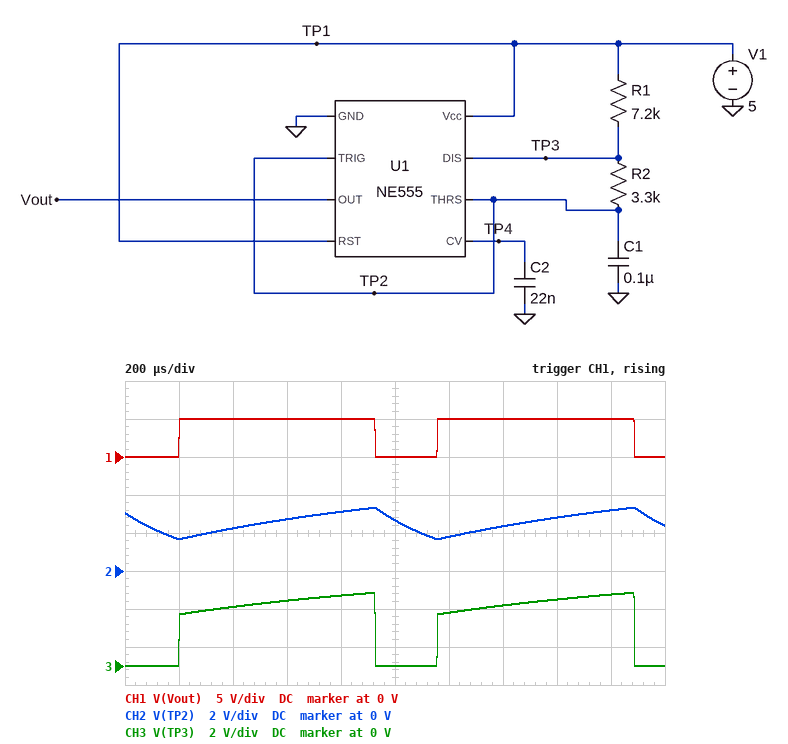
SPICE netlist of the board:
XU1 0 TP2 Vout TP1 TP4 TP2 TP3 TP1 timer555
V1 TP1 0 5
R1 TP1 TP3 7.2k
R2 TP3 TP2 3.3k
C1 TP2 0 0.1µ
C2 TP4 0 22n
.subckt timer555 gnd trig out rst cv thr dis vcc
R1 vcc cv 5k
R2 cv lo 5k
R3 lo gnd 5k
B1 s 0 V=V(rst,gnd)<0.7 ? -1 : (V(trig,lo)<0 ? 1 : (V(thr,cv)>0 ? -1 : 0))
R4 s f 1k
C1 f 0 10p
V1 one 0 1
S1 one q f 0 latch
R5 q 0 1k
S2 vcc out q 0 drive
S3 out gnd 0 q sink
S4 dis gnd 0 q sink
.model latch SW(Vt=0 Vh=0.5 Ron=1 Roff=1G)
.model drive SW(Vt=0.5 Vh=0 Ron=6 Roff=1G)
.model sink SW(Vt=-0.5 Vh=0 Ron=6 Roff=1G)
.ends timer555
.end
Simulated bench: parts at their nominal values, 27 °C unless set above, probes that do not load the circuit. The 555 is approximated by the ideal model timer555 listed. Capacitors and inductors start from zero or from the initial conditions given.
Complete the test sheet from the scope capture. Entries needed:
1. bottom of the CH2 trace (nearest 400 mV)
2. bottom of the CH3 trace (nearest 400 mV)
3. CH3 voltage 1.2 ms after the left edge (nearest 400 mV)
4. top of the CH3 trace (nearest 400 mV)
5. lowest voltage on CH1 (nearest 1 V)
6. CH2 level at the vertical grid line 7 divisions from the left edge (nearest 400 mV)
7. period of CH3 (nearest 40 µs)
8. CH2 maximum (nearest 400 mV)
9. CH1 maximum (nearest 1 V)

1.6 V
0 V
2.8 V
4.0 V
0 V
2.4 V
960 µs
3.2 V
5 V
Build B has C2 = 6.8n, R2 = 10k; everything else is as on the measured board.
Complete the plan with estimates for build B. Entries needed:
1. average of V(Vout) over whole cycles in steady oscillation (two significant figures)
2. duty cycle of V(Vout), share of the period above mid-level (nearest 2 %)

3.2 V
64 %
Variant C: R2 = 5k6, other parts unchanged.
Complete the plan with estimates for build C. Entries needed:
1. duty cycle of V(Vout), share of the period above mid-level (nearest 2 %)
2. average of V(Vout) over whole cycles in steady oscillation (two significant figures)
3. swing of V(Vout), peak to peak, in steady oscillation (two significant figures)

70 %
3.5 V
5.0 V
